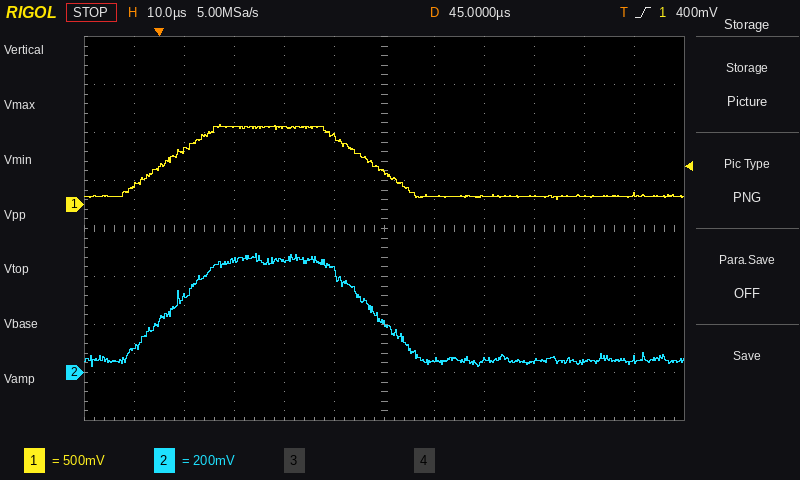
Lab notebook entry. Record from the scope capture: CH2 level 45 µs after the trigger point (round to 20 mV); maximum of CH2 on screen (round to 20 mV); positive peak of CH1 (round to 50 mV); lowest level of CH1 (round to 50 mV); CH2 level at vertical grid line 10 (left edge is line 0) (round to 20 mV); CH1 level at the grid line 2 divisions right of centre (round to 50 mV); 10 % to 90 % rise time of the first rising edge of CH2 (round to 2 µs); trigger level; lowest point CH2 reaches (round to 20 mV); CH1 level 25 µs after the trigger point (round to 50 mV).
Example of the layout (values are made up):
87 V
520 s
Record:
200 mV
500 mV
850 mV
50 mV
40 mV
100 mV
16 µs
400 mV
20 mV
800 mV
